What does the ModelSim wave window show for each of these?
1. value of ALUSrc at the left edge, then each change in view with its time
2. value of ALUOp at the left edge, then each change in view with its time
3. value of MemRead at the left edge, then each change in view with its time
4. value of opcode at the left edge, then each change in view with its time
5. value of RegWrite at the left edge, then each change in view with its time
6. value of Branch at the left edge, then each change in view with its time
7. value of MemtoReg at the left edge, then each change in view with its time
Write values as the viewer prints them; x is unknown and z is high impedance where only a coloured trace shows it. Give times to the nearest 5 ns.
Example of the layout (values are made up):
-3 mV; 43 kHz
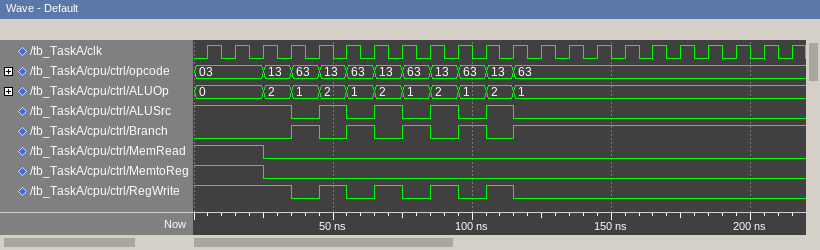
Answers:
1, 0 at 35 ns, 1 at 45 ns, 0 at 55 ns, 1 at 65 ns, 0 at 75 ns, 1 at 85 ns, 0 at 95 ns, 1 at 105 ns, 0 at 115 ns; 0, 2 at 25 ns, 1 at 35 ns, 2 at 45 ns, 1 at 55 ns, 2 at 65 ns, 1 at 75 ns, 2 at 85 ns, 1 at 95 ns, 2 at 105 ns, 1 at 115 ns; 1, 0 at 25 ns; 03, 13 at 25 ns, 63 at 35 ns, 13 at 45 ns, 63 at 55 ns, 13 at 65 ns, 63 at 75 ns, 13 at 85 ns, 63 at 95 ns, 13 at 105 ns, 63 at 115 ns; 1, 0 at 35 ns, 1 at 45 ns, 0 at 55 ns, 1 at 65 ns, 0 at 75 ns, 1 at 85 ns, 0 at 95 ns, 1 at 105 ns, 0 at 115 ns; 0, 1 at 35 ns, 0 at 45 ns, 1 at 55 ns, 0 at 65 ns, 1 at 75 ns, 0 at 85 ns, 1 at 95 ns, 0 at 105 ns, 1 at 115 ns; 1, 0 at 25 ns
